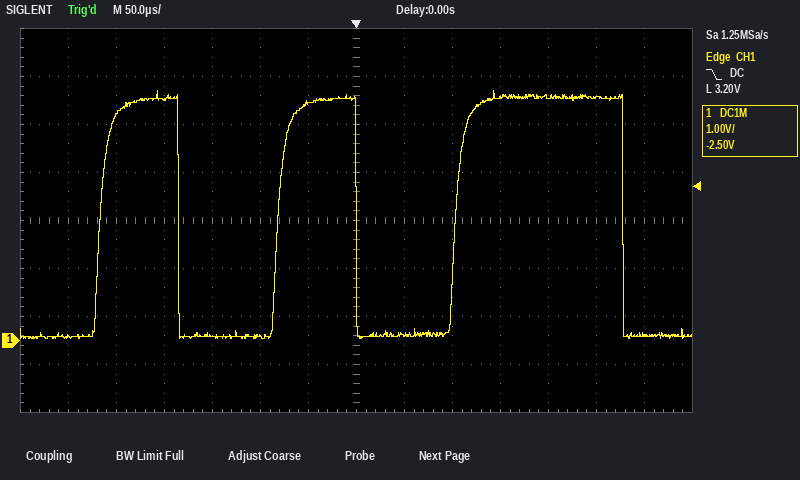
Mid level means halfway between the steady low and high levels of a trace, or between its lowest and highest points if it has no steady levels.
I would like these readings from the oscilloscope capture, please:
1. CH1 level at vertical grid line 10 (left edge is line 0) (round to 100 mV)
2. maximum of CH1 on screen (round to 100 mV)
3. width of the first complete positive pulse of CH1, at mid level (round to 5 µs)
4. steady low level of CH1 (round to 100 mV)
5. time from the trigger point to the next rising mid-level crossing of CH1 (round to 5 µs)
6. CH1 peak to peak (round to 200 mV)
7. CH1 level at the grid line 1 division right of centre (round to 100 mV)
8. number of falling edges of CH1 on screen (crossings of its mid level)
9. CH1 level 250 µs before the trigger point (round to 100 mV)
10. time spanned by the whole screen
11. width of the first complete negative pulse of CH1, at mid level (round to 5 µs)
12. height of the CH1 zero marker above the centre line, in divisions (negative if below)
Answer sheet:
5.1 V
5.2 V
80 µs
100 mV
105 µs
5.2 V
100 mV
3
4.7 V
700 µs
105 µs
-2.5 div
